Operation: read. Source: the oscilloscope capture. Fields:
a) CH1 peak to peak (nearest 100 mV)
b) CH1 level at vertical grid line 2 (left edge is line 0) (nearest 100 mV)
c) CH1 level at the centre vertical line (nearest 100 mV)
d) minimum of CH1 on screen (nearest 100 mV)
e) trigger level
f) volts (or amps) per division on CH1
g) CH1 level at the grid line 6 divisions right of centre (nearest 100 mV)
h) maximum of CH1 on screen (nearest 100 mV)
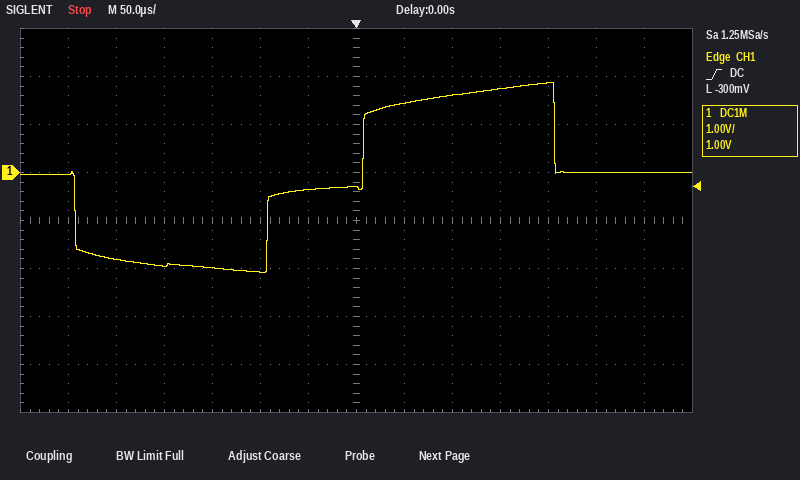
4.0 V
-1.8 V
-300 mV
-2.1 V
-300 mV
1 V
0.0 V
1.9 V
